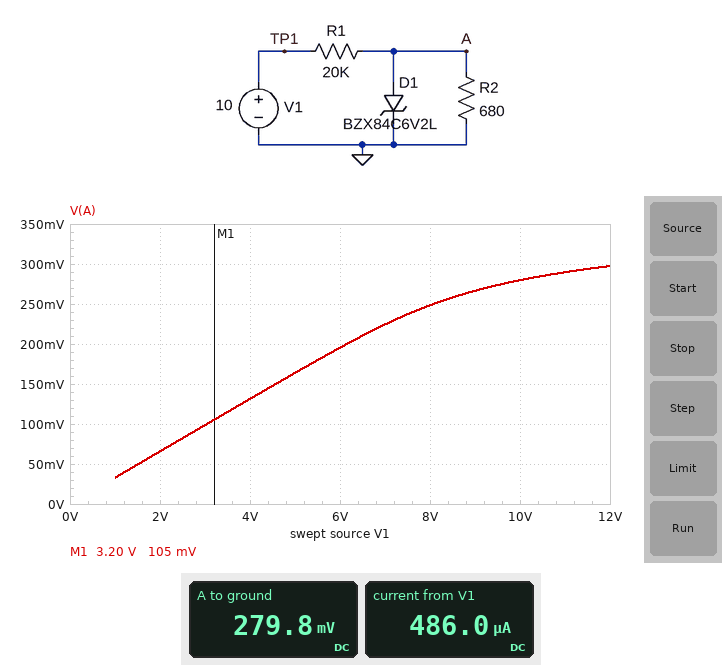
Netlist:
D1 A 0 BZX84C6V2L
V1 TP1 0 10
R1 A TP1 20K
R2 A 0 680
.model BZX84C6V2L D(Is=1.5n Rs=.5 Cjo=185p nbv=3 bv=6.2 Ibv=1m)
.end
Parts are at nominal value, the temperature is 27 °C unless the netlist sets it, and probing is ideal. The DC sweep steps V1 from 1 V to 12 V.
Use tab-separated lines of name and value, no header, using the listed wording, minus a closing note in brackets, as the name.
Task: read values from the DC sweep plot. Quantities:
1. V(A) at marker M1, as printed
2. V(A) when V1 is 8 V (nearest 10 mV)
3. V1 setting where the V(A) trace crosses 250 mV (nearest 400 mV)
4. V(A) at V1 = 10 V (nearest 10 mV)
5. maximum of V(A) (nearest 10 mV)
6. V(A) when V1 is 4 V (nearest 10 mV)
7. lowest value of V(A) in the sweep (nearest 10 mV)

V(A) at marker M1, as printed	105 mV
V(A) when V1 is 8 V	250 mV
V1 setting where the V(A) trace crosses 250 mV	8.0 V
V(A) at V1 = 10 V	280 mV
maximum of V(A)	300 mV
V(A) when V1 is 4 V	130 mV
lowest value of V(A) in the sweep	30 mV
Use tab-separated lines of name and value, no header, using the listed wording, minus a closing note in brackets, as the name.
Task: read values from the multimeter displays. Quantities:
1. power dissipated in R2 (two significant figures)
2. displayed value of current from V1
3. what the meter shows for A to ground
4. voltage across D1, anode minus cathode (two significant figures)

power dissipated in R2	120 µW
displayed value of current from V1	486.0 µA
what the meter shows for A to ground	279.8 mV
voltage across D1, anode minus cathode	280 mV
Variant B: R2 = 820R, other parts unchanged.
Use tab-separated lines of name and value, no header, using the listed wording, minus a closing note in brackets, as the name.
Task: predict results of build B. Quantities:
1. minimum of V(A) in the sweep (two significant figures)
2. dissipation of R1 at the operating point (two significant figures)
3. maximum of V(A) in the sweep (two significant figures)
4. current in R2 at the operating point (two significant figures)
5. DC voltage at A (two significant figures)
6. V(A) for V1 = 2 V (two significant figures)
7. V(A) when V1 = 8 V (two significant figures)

minimum of V(A) in the sweep	39 mV
dissipation of R1 at the operating point	4.7 mW
maximum of V(A) in the sweep	310 mV
current in R2 at the operating point	360 µA
DC voltage at A	290 mV
V(A) for V1 = 2 V	79 mV
V(A) when V1 = 8 V	270 mV
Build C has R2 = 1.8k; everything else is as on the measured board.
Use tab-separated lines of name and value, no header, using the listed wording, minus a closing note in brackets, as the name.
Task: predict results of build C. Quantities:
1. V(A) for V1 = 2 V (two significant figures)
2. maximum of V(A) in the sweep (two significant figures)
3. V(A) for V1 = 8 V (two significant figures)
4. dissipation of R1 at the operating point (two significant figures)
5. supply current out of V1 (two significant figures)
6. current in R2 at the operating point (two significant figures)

V(A) for V1 = 2 V	160 mV
maximum of V(A) in the sweep	320 mV
V(A) for V1 = 8 V	310 mV
dissipation of R1 at the operating point	4.7 mW
supply current out of V1	480 µA
current in R2 at the operating point	180 µA
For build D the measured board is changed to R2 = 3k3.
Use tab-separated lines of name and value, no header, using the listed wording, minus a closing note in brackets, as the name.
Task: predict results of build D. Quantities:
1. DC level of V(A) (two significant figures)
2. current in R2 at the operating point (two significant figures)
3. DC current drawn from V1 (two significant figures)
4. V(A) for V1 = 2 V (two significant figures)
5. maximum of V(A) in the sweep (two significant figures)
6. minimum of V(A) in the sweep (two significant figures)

DC level of V(A)	320 mV
current in R2 at the operating point	98 µA
DC current drawn from V1	480 µA
V(A) for V1 = 2 V	240 mV
maximum of V(A) in the sweep	330 mV
minimum of V(A) in the sweep	140 mV
